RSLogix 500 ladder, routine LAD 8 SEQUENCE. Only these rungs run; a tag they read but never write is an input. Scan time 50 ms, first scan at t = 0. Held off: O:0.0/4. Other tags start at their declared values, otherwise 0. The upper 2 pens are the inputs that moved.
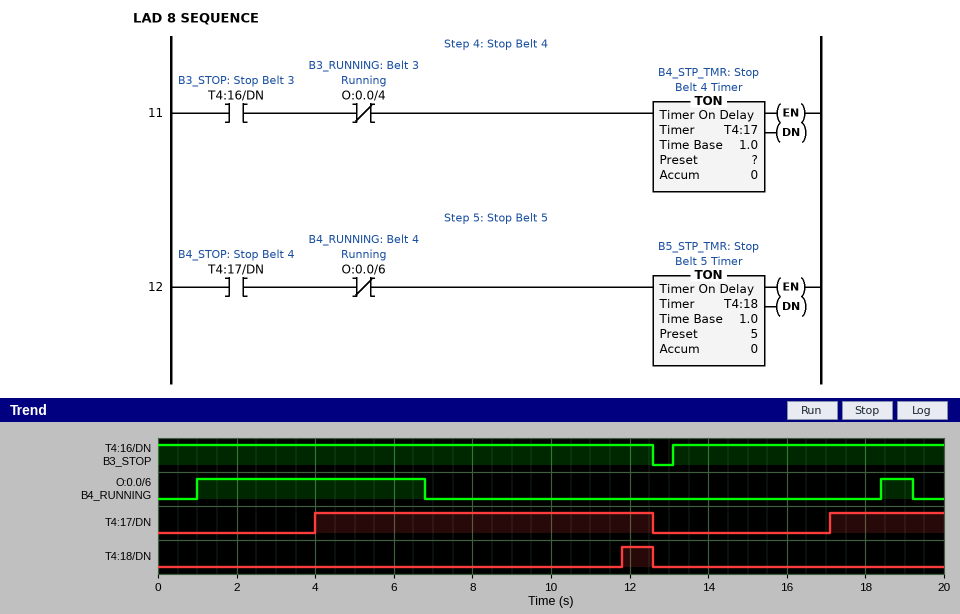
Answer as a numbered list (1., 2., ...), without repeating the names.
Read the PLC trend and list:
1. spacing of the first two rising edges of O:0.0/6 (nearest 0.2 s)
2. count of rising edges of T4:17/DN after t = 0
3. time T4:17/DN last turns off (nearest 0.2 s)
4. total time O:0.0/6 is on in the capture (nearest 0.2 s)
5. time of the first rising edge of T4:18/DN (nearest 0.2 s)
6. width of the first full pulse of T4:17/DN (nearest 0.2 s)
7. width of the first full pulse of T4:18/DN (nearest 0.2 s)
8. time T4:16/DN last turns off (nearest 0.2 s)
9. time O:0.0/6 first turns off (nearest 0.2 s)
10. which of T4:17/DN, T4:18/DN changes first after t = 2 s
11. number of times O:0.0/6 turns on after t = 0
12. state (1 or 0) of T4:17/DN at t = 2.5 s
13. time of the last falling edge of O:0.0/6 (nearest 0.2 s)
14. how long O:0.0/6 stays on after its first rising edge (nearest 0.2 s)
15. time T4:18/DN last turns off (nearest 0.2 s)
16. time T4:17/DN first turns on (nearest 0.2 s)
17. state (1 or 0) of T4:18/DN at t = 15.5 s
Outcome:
1. 17.4 s
2. 2
3. 12.6 s
4. 6.6 s
5. 11.8 s
6. 8.6 s
7. 0.8 s
8. 12.6 s
9. 6.8 s
10. T4:17/DN
11. 2
12. 0
13. 19.2 s
14. 5.8 s
15. 12.6 s
16. 4.0 s
17. 0
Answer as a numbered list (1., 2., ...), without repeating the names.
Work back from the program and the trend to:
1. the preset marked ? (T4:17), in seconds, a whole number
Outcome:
1. 4 s
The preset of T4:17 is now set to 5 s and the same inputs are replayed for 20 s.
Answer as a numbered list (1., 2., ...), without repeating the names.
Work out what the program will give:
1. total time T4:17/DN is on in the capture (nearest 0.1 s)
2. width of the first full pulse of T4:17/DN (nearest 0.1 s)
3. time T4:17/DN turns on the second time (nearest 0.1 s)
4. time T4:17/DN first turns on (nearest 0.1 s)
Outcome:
1. 9.5 s
2. 7.6 s
3. 18.1 s
4. 5.0 s
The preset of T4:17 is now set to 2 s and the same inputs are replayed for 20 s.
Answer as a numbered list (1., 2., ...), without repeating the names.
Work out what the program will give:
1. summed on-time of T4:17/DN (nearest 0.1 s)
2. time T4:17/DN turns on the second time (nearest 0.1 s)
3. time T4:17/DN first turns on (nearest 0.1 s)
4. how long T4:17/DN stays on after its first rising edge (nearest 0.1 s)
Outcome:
1. 15.5 s
2. 15.1 s
3. 2.0 s
4. 10.6 s
